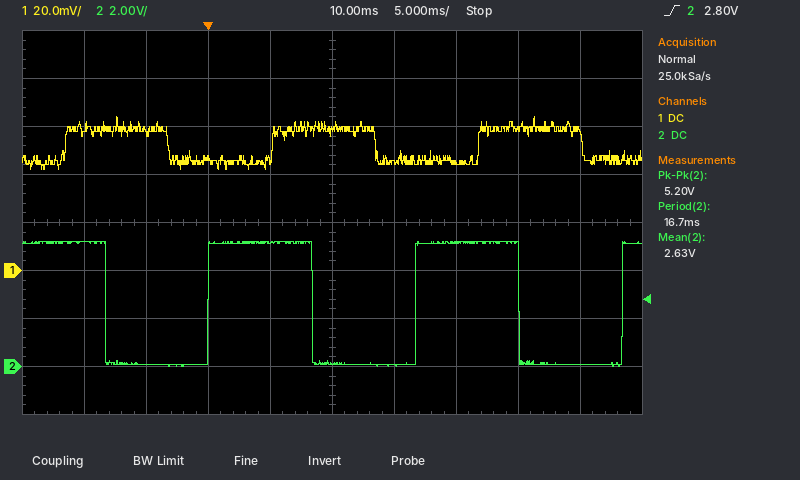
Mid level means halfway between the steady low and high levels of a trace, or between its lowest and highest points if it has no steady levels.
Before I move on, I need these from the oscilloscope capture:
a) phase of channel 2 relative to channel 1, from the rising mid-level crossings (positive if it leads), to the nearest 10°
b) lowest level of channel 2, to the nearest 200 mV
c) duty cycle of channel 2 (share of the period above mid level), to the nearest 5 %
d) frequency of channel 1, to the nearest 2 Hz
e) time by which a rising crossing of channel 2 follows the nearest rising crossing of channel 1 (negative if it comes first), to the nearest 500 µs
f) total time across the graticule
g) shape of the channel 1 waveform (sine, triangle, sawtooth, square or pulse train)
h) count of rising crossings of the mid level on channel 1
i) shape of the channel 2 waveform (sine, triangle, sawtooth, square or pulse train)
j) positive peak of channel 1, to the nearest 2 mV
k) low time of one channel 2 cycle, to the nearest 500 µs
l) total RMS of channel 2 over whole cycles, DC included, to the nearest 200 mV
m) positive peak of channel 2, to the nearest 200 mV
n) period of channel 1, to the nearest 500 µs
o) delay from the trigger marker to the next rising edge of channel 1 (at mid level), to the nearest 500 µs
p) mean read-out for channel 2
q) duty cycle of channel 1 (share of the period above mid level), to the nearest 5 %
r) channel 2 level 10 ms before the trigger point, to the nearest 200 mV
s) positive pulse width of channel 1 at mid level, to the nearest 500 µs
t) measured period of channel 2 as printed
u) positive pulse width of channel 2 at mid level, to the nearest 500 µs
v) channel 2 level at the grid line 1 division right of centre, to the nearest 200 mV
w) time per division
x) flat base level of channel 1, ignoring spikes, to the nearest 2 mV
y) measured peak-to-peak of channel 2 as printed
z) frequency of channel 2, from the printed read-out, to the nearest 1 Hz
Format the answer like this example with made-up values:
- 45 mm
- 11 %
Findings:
- +110°
- 0.0 V
- 50 %
- 60 Hz
- -5.0 ms
- 50 ms
- square
- 3
- square
- 64 mV
- 8.5 ms
- 3.6 V
- 5.2 V
- 16.5 ms
- 5.0 ms
- 2.63 V
- 50 %
- 5.2 V
- 8.5 ms
- 16.7 ms
- 8.5 ms
- 0.0 V
- 5 ms
- 46 mV
- 5.20 V
- 60 Hz
